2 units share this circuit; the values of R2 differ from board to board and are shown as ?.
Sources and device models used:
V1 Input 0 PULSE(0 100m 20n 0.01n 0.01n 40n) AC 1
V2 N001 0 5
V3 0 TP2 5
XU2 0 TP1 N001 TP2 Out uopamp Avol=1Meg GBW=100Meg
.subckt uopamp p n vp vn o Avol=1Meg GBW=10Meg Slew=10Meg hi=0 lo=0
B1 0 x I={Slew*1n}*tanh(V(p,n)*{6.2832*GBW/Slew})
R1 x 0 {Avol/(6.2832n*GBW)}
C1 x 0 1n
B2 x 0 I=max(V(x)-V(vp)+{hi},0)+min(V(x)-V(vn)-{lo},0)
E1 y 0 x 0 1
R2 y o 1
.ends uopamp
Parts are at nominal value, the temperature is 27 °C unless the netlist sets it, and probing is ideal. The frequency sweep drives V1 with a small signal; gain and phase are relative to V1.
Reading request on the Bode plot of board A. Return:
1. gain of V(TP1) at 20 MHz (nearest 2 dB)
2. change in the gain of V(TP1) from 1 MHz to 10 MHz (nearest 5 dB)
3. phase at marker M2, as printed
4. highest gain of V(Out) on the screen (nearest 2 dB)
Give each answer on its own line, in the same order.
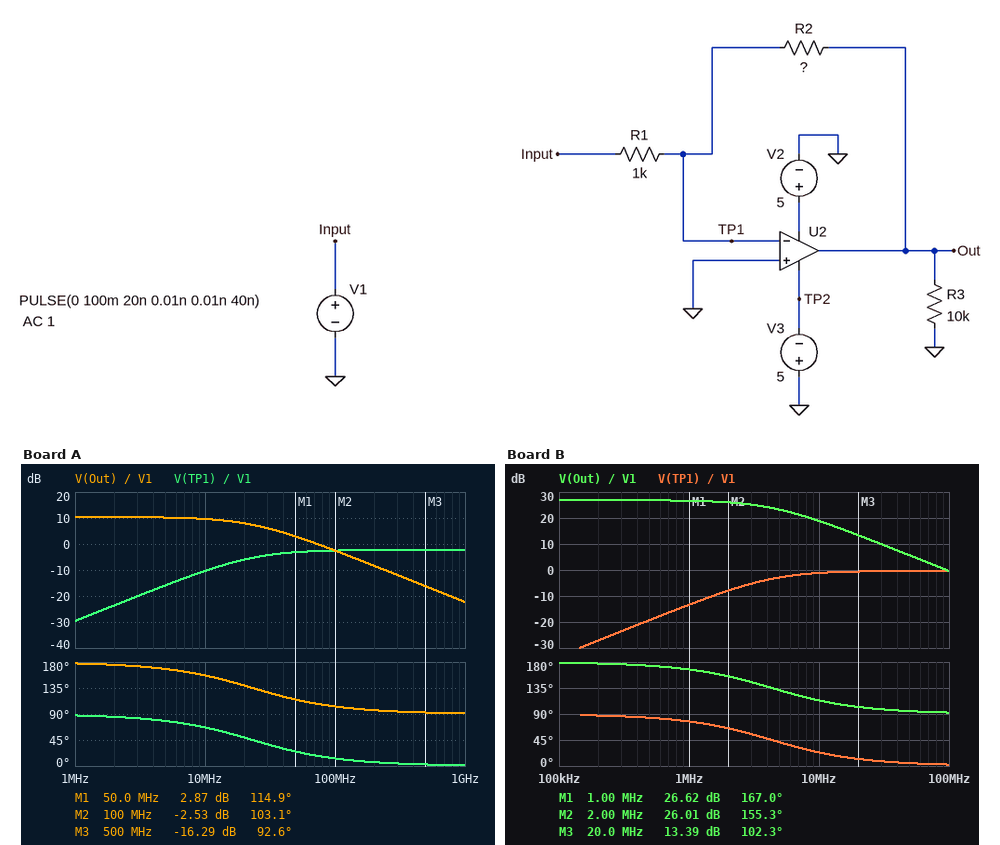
-6 dB
20 dB
103.1 deg
10 dB
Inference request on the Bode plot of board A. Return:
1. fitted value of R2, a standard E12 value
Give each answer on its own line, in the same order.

3.3 kΩ
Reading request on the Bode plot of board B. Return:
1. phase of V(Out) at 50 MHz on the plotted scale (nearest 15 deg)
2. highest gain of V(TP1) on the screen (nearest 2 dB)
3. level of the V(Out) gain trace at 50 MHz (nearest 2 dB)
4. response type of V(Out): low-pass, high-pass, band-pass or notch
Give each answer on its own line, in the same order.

90 deg
0 dB
6 dB
low-pass
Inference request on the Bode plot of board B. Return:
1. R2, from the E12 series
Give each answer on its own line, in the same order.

22 kΩ
